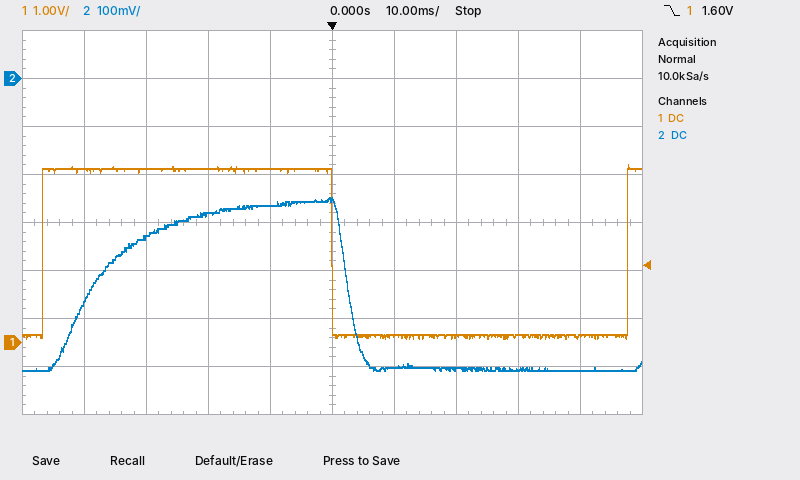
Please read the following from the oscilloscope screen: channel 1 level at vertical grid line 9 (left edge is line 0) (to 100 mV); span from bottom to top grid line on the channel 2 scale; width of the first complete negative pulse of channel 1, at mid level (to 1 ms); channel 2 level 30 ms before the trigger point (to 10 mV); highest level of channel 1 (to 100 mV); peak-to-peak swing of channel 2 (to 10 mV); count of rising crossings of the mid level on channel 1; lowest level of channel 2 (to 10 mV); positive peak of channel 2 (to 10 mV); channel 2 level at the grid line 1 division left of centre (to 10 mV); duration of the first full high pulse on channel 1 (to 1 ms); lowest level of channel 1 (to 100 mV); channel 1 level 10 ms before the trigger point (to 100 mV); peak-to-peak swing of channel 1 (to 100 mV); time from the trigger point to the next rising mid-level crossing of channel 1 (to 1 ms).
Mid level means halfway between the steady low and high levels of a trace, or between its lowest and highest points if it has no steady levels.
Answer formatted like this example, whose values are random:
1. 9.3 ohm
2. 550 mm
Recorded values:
1. 100 mV
2. 800 mV
3. 48 ms
4. -330 mV
5. 3.7 V
6. 360 mV
7. 2
8. -610 mV
9. -250 mV
10. -260 mV
11. 47 ms
12. 100 mV
13. 3.6 V
14. 3.6 V
15. 48 ms
